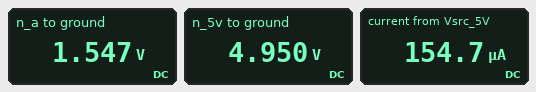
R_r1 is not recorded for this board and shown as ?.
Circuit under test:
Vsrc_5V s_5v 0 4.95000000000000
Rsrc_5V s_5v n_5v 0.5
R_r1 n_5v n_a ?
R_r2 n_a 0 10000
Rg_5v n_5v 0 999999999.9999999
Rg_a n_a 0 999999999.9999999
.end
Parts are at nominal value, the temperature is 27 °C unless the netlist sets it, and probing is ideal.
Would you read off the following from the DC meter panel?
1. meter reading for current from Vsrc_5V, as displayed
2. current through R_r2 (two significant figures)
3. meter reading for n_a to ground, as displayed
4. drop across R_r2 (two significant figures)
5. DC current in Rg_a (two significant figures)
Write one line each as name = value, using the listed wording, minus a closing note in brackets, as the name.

meter reading for current from Vsrc_5V, as displayed = 154.7 µA
current through R_r2 = 150 µA
meter reading for n_a to ground, as displayed = 1.547 V
drop across R_r2 = 1.5 V
DC current in Rg_a = 1.5 nA
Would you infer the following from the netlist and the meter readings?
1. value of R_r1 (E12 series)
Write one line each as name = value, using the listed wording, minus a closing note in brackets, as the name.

value of R_r1 = 22 kΩ
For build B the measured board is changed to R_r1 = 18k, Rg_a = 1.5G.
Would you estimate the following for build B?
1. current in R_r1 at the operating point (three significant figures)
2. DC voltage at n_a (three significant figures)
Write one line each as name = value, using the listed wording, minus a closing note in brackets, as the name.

current in R_r1 at the operating point = 177 µA
DC voltage at n_a = 1.77 V
